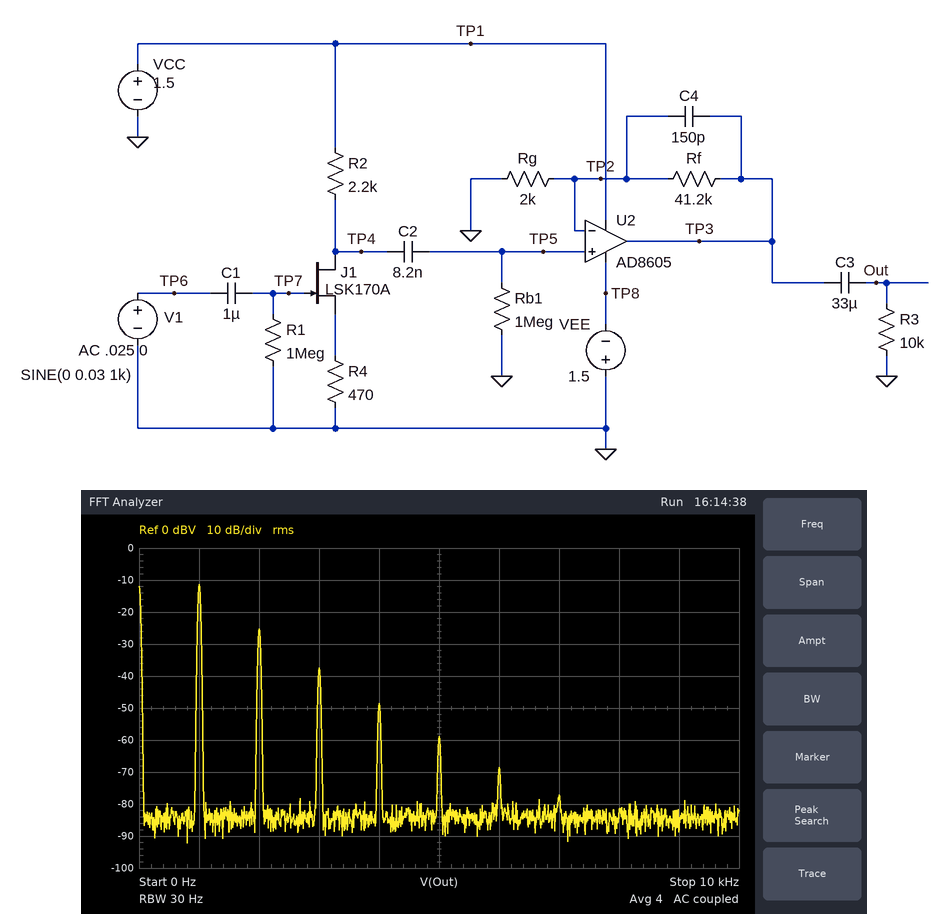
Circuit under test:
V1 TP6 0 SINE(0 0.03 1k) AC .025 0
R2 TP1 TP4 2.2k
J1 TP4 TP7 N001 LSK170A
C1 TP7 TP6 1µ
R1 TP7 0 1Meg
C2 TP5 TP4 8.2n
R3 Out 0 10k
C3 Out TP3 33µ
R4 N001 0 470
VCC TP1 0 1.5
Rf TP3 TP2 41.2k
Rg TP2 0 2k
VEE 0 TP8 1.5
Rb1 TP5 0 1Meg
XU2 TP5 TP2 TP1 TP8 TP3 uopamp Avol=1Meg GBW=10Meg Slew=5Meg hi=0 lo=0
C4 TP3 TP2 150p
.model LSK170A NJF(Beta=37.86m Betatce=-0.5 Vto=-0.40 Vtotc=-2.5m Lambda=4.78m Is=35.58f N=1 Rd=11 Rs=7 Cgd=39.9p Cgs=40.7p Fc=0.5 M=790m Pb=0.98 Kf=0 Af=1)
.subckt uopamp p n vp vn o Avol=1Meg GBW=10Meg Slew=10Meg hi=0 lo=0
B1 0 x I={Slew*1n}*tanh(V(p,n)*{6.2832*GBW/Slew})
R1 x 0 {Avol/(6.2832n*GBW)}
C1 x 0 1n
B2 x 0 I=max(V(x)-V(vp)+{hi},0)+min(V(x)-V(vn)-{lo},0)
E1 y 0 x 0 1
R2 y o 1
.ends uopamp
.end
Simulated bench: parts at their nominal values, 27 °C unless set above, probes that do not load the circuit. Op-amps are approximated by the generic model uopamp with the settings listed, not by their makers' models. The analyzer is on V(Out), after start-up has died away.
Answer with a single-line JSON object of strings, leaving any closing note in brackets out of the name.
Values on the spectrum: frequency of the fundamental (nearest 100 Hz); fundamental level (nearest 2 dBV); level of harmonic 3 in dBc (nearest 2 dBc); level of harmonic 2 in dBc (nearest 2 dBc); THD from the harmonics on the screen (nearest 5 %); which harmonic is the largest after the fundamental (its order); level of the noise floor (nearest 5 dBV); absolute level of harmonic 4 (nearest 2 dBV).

{"frequency of the fundamental": "1.0 kHz", "fundamental level": "-12 dBV", "level of harmonic 3 in dBc": "-26 dBc", "level of harmonic 2 in dBc": "-14 dBc", "THD from the harmonics on the screen": "20 %", "which harmonic is the largest after the fundamental": "2", "level of the noise floor": "-85 dBV", "absolute level of harmonic 4": "-48 dBV"}
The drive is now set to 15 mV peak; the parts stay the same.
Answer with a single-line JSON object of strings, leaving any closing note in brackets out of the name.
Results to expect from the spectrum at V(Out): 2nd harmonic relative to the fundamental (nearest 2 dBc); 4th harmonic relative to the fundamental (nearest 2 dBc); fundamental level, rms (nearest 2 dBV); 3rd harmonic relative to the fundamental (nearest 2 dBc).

{"2nd harmonic relative to the fundamental": "-20 dBc", "4th harmonic relative to the fundamental": "-58 dBc", "fundamental level, rms": "-18 dBV", "3rd harmonic relative to the fundamental": "-40 dBc"}
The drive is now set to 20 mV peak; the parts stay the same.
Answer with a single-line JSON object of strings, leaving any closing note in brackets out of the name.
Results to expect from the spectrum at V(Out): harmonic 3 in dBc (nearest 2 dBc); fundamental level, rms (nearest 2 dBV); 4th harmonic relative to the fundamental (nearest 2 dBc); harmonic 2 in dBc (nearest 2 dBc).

{"harmonic 3 in dBc": "-34 dBc", "fundamental level, rms": "-16 dBV", "4th harmonic relative to the fundamental": "-50 dBc", "harmonic 2 in dBc": "-18 dBc"}
